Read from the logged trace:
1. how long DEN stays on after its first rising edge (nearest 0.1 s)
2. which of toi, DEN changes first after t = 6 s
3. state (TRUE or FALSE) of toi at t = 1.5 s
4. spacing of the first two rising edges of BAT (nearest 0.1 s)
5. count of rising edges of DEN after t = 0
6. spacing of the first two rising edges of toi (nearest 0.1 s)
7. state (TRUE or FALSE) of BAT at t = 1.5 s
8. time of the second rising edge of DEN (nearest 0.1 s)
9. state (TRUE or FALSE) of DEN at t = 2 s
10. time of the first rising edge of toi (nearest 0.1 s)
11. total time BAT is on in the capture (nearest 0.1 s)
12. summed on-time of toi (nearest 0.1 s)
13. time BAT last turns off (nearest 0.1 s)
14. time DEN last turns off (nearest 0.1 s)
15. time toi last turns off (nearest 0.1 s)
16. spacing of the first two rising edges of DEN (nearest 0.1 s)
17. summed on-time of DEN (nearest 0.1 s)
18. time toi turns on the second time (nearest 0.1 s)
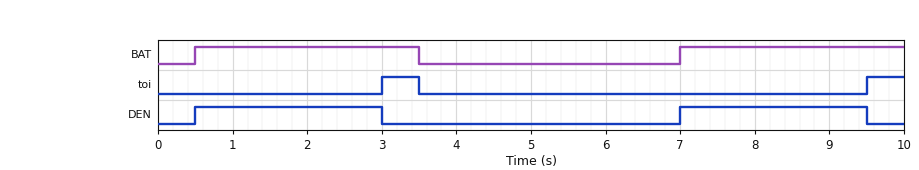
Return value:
2.5 s
DEN
FALSE
6.5 s
2
6.5 s
TRUE
7.0 s
TRUE
3.0 s
6.0 s
1.0 s
3.5 s
9.5 s
3.5 s
6.5 s
5.0 s
9.5 s
